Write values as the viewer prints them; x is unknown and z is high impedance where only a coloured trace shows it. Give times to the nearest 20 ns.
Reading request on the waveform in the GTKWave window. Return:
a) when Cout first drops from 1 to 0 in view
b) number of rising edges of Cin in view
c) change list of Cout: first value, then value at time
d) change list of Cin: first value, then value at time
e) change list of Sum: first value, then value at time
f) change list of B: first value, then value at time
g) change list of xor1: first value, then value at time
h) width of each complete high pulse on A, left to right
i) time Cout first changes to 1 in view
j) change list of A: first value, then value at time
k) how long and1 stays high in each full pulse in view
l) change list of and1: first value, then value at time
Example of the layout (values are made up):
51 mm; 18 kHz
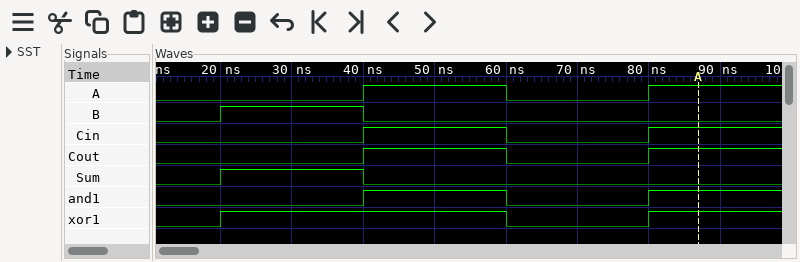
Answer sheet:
60 ns; 2; 0, 1 at 40 ns, 0 at 60 ns, 1 at 80 ns; 0, 1 at 40 ns, 0 at 60 ns, 1 at 80 ns; 0, 1 at 20 ns, 0 at 40 ns; 0, 1 at 20 ns, 0 at 40 ns; 0, 1 at 20 ns, 0 at 60 ns, 1 at 80 ns; 20 ns; 40 ns; 0, 1 at 40 ns, 0 at 60 ns, 1 at 80 ns; 20 ns; 0, 1 at 40 ns, 0 at 60 ns, 1 at 80 ns
